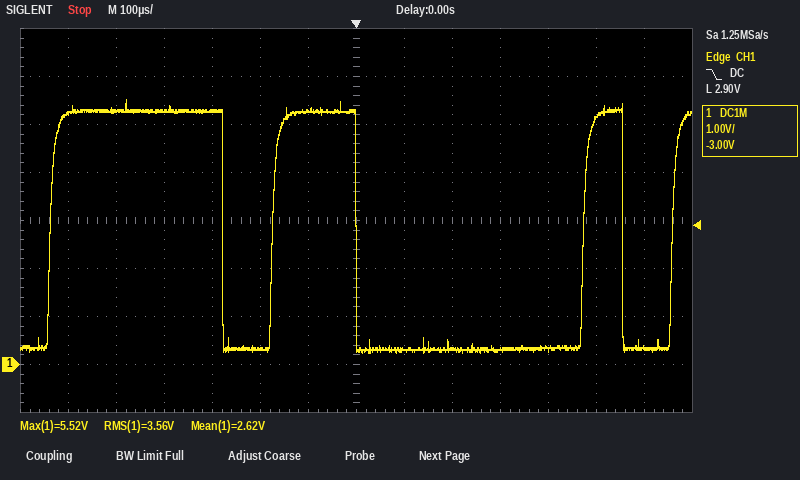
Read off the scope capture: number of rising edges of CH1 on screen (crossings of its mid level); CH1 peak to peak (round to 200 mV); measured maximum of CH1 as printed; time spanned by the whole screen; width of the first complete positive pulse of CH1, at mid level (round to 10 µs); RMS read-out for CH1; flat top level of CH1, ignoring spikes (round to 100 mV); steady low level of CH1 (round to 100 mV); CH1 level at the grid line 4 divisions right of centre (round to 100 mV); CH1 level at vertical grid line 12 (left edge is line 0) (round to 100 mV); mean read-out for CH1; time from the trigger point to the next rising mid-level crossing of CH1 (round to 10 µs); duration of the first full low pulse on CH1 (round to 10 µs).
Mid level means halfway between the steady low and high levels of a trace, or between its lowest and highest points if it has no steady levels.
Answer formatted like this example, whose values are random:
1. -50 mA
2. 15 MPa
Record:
1. 4
2. 5.2 V
3. 5.52 V
4. 1.4 ms
5. 360 µs
6. 3.56 V
7. 5.3 V
8. 300 mV
9. 300 mV
10. 5.1 V
11. 2.62 V
12. 470 µs
13. 100 µs
